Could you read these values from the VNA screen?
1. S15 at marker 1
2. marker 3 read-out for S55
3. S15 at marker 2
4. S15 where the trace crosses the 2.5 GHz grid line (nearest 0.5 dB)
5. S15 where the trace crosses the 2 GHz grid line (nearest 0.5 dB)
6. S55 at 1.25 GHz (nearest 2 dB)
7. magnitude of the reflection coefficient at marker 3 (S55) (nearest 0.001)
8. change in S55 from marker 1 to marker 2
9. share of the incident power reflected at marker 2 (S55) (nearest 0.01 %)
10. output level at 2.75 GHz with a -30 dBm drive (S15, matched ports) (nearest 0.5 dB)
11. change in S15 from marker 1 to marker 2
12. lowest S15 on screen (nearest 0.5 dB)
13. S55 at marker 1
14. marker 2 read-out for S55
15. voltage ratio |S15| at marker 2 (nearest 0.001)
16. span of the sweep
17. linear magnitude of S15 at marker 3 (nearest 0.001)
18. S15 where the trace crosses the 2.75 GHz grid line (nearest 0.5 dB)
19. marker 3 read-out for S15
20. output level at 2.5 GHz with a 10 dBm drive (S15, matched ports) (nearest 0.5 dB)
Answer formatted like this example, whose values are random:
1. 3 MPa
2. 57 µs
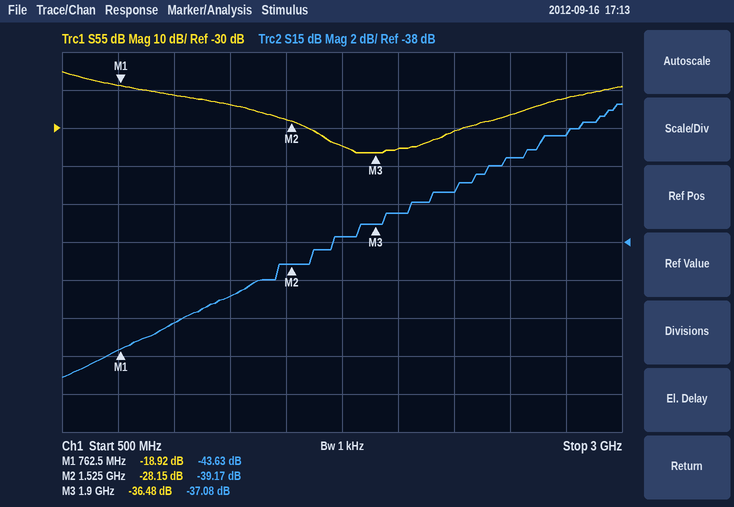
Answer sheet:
1. -43.63 dB
2. -36.48 dB
3. -39.17 dB
4. -33.5 dB
5. -36.5 dB
6. -24 dB
7. 0.015
8. -9.23 dB
9. 0.15 %
10. -62.5 dBm
11. 4.46 dB
12. -45.0 dB
13. -18.92 dB
14. -28.15 dB
15. 0.011
16. 2.5 GHz
17. 0.014
18. -32.5 dB
19. -37.08 dB
20. -23.5 dBm
